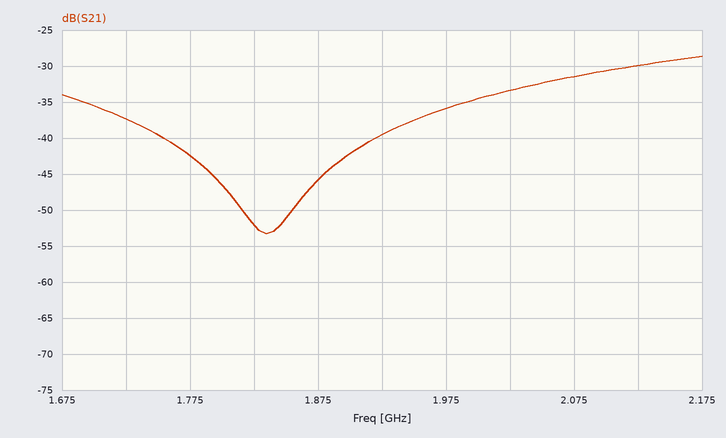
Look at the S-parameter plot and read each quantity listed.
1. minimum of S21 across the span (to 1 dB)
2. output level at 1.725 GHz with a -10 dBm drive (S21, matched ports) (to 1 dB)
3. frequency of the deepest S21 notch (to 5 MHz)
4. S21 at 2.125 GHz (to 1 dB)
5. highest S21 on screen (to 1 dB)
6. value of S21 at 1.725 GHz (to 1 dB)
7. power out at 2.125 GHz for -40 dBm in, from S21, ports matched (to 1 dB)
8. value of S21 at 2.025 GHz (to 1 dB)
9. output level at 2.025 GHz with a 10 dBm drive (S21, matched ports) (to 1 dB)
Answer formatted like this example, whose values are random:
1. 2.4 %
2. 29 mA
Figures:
1. -53 dB
2. -47 dBm
3. 1.835 GHz
4. -30 dB
5. -29 dB
6. -37 dB
7. -70 dBm
8. -33 dB
9. -23 dBm
